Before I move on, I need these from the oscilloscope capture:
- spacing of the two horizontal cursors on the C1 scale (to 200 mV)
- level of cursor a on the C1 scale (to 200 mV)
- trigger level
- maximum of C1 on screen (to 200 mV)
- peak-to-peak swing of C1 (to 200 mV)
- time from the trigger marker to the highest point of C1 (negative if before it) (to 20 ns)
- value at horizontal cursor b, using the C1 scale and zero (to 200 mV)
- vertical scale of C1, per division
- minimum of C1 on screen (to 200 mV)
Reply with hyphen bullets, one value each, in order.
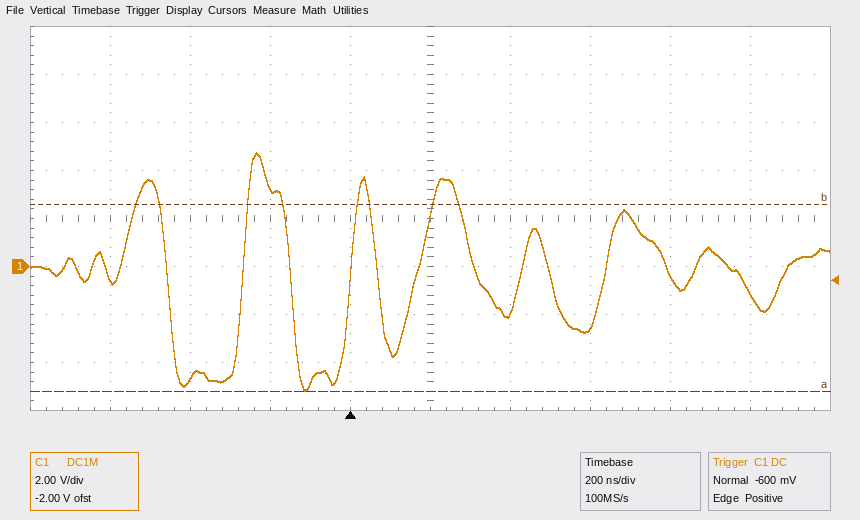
- 7.8 V
- -5.2 V
- -600 mV
- 4.8 V
- 10.0 V
- -240 ns
- 2.6 V
- 2 V
- -5.2 V
